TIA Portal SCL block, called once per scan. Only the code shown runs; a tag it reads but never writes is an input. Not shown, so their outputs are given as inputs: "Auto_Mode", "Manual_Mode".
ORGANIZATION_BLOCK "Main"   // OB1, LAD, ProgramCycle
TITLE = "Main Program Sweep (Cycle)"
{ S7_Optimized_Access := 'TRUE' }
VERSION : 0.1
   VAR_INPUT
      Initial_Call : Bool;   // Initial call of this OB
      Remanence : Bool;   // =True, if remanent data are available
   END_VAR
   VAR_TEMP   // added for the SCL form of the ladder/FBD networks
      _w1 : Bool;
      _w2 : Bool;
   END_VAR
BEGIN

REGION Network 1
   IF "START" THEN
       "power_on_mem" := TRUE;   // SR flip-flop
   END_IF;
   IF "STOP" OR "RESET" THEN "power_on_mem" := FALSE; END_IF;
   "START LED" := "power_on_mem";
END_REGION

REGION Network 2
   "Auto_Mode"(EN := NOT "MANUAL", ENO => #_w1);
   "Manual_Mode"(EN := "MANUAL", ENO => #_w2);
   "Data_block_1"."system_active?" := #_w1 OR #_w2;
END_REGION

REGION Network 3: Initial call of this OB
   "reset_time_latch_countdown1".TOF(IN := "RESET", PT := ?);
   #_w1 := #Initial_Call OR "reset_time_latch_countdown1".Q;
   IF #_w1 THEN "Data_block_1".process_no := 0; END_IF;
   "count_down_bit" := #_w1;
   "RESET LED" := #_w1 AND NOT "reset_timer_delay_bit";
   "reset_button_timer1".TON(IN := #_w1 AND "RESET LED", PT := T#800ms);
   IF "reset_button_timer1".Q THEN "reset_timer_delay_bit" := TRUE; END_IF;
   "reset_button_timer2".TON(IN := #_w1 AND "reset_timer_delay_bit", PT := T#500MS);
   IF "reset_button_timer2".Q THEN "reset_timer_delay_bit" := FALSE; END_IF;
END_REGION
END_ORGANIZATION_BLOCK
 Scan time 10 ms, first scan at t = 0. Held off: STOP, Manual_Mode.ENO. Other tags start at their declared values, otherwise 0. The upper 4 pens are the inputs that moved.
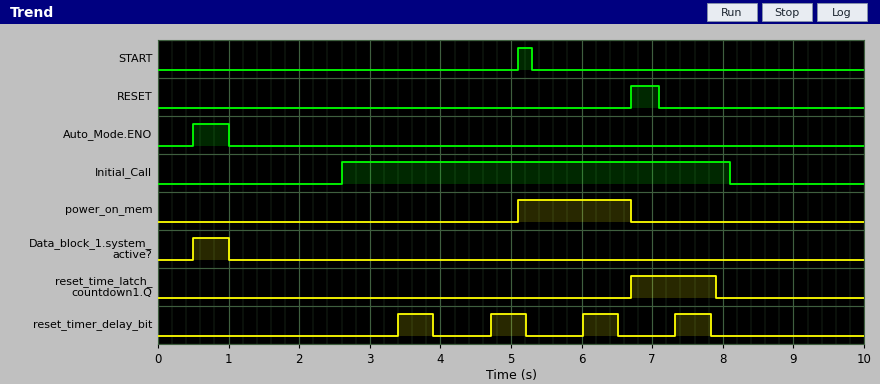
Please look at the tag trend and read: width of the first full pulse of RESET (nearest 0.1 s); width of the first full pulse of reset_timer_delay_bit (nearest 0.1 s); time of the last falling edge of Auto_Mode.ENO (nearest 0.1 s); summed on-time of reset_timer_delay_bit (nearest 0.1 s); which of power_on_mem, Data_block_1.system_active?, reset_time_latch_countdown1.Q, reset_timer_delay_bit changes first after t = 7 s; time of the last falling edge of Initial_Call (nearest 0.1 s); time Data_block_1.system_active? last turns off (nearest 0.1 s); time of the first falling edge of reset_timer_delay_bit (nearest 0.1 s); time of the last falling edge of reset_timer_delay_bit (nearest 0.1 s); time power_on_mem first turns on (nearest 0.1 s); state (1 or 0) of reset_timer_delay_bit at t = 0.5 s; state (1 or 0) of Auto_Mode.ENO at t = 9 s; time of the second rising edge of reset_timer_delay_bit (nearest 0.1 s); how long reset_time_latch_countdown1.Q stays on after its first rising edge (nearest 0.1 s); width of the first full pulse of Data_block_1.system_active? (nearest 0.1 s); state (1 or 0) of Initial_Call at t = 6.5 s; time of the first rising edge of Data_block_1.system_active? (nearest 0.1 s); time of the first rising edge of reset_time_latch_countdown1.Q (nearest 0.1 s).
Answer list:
0.4 s
0.5 s
1.0 s
2.0 s
reset_timer_delay_bit
8.1 s
1.0 s
3.9 s
7.8 s
5.1 s
0
0
4.7 s
1.2 s
0.5 s
1
0.5 s
6.7 s
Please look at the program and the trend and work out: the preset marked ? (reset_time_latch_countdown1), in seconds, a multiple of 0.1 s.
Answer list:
0.8 s
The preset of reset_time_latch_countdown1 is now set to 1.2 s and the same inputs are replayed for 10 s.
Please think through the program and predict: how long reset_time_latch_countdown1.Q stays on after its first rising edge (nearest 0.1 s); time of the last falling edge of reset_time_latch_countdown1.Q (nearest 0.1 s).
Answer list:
1.6 s
8.3 s
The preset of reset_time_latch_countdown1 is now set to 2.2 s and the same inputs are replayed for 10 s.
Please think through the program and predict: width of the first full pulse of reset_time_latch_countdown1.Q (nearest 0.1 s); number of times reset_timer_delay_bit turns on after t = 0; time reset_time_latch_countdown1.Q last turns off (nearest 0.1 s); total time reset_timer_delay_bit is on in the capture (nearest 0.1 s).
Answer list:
2.6 s
5
9.3 s
2.5 s
